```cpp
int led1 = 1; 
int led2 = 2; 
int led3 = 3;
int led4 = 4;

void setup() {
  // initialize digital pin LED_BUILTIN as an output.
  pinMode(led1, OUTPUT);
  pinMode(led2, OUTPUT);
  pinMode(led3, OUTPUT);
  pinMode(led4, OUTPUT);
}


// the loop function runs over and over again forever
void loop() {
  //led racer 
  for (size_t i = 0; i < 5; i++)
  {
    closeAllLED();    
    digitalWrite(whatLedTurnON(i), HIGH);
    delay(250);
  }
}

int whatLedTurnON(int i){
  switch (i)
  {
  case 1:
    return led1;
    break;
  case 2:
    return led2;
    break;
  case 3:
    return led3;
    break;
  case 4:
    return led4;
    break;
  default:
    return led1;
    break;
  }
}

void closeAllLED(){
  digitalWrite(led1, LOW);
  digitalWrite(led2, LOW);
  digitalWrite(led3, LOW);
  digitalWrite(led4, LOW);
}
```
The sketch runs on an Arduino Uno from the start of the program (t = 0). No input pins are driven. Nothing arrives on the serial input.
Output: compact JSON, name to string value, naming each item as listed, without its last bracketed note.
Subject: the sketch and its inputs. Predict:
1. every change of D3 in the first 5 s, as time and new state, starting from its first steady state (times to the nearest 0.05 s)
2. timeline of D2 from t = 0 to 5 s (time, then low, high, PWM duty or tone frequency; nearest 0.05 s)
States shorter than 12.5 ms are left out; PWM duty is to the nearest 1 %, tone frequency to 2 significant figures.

{"every change of D3 in the first 5 s, as time and new state, starting from its first steady state": "0 s low; 0.75 s high; 1 s low; 2 s high; 2.25 s low; 3.25 s high; 3.5 s low; 4.5 s high; 4.75 s low", "timeline of D2 from t = 0 to 5 s": "0 s low; 0.5 s high; 0.75 s low; 1.75 s high; 2 s low; 3 s high; 3.25 s low; 4.25 s high; 4.5 s low"}
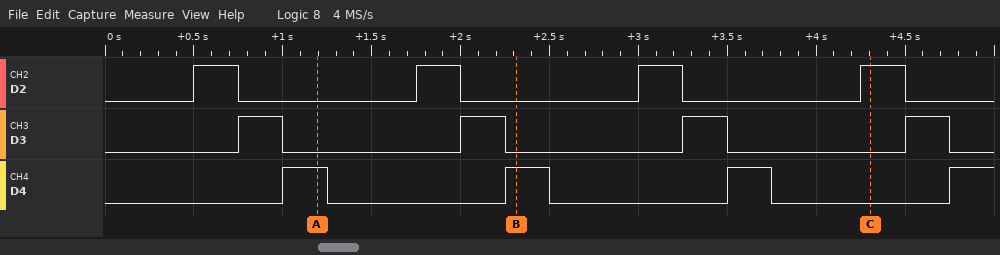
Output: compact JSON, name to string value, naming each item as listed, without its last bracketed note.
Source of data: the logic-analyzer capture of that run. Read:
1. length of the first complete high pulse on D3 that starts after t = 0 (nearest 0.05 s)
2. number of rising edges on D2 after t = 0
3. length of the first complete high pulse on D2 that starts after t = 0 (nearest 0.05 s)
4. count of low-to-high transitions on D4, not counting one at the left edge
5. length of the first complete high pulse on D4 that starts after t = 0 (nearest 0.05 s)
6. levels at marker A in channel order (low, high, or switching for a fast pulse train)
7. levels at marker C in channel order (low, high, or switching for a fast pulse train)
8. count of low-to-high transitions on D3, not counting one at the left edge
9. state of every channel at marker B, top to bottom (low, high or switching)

{"length of the first complete high pulse on D3 that starts after t = 0": "0.25 s", "number of rising edges on D2 after t = 0": "4", "length of the first complete high pulse on D2 that starts after t = 0": "0.25 s", "count of low-to-high transitions on D4, not counting one at the left edge": "4", "length of the first complete high pulse on D4 that starts after t = 0": "0.25 s", "levels at marker A in channel order": "D2 low, D3 low, D4 high", "levels at marker C in channel order": "D2 high, D3 low, D4 low", "count of low-to-high transitions on D3, not counting one at the left edge": "4", "state of every channel at marker B, top to bottom": "D2 low, D3 low, D4 high"}
